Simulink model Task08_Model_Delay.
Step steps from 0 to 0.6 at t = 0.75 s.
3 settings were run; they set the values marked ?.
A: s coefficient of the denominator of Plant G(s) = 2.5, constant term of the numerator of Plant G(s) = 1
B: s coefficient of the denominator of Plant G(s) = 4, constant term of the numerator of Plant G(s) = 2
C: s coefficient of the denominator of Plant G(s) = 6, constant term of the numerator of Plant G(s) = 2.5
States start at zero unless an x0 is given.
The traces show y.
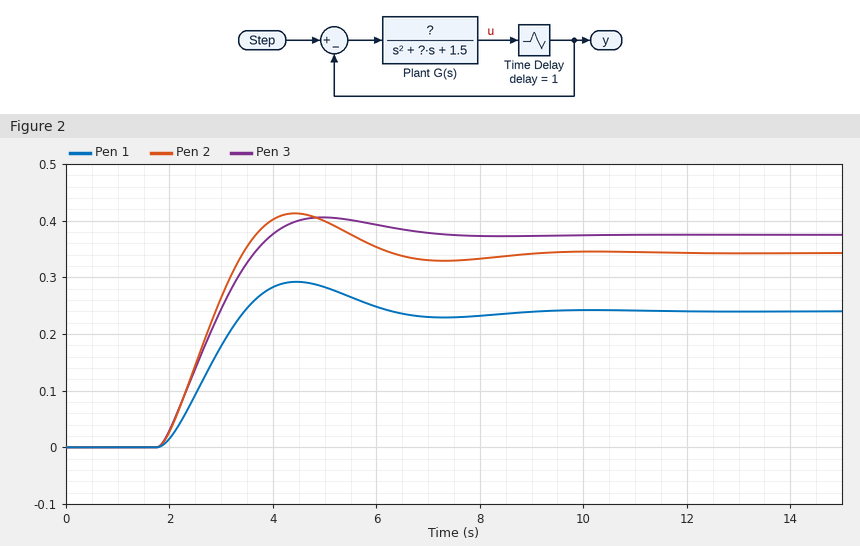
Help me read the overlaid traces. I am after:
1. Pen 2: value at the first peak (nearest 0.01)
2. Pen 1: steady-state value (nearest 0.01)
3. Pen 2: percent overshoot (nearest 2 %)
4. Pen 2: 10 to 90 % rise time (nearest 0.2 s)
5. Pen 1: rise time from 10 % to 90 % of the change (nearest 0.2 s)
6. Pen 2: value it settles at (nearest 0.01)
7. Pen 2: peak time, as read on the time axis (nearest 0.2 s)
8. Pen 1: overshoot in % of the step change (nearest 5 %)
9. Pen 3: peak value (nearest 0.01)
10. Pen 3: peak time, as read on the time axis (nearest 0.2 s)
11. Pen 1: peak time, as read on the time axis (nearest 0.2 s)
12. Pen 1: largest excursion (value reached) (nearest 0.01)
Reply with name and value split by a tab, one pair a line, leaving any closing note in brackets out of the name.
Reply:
Pen 2: value at the first peak	0.41
Pen 1: steady-state value	0.24
Pen 2: percent overshoot	20 %
Pen 2: 10 to 90 % rise time	1.2 s
Pen 1: rise time from 10 % to 90 % of the change	1.2 s
Pen 2: value it settles at	0.34
Pen 2: peak time, as read on the time axis	4.4 s
Pen 1: overshoot in % of the step change	20 %
Pen 3: peak value	0.41
Pen 3: peak time, as read on the time axis	5.0 s
Pen 1: peak time, as read on the time axis	4.4 s
Pen 1: largest excursion (value reached)	0.29
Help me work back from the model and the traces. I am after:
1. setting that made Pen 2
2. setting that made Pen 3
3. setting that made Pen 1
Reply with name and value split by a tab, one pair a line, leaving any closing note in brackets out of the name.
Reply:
setting that made Pen 2	B
setting that made Pen 3	C
setting that made Pen 1	A
